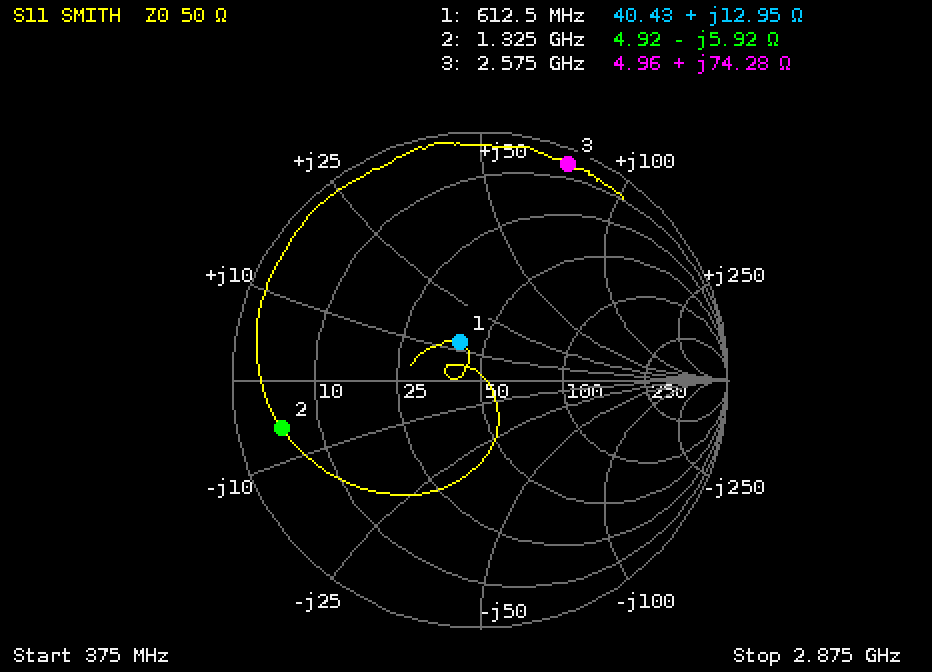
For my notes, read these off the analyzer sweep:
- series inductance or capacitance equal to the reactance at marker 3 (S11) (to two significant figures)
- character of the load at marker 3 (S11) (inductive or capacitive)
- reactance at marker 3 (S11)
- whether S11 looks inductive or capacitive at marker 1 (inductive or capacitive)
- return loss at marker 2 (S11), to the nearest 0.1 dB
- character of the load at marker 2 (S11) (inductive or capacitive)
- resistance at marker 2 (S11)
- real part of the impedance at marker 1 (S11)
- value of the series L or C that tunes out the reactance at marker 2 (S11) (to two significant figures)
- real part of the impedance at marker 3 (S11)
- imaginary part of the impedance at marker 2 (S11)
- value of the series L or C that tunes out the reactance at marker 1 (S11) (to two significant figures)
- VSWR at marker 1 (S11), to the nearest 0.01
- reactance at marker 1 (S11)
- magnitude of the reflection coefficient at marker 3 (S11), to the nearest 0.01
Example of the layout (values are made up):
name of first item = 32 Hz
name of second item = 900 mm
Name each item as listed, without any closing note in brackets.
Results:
series inductance or capacitance equal to the reactance at marker 3 (S11) = 4.6 nH
character of the load at marker 3 (S11) = inductive
reactance at marker 3 = +74.28 Ω
whether S11 looks inductive or capacitive at marker 1 = inductive
return loss at marker 2 (S11), to the nearest 0.1 dB = 1.7 dB
character of the load at marker 2 (S11) = capacitive
resistance at marker 2 = 4.92 Ω
real part of the impedance at marker 1 = 40.43 Ω
value of the series L or C that tunes out the reactance at marker 2 (S11) = 710 pH
real part of the impedance at marker 3 = 4.96 Ω
imaginary part of the impedance at marker 2 = -5.92 Ω
value of the series L or C that tunes out the reactance at marker 1 (S11) = 20 pF
VSWR at marker 1 (S11), to the nearest 0.01 = 1.43
reactance at marker 1 = +12.95 Ω
magnitude of the reflection coefficient at marker 3 (S11), to the nearest 0.01 = 0.94
